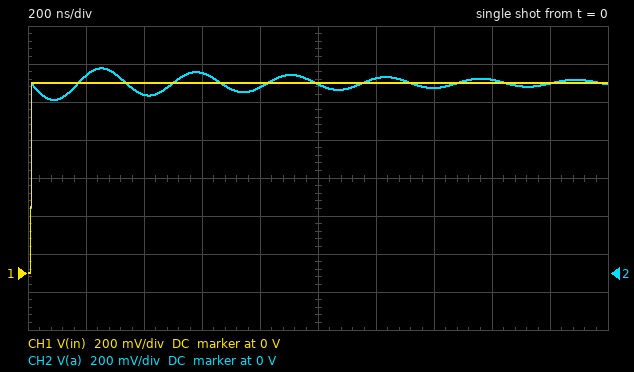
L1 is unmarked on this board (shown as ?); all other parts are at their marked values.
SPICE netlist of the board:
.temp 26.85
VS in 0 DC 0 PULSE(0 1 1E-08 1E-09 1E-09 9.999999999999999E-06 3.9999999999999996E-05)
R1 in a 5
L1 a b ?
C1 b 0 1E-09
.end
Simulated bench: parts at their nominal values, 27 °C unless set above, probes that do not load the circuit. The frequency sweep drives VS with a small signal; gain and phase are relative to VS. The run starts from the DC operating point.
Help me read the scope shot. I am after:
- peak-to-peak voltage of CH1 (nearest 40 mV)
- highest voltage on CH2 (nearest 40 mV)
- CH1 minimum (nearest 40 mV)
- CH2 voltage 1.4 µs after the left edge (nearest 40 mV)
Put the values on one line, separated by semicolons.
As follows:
1.00 V; 1.08 V; 0 V; 960 mV
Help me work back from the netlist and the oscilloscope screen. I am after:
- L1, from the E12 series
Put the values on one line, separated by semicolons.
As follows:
2.7 µH
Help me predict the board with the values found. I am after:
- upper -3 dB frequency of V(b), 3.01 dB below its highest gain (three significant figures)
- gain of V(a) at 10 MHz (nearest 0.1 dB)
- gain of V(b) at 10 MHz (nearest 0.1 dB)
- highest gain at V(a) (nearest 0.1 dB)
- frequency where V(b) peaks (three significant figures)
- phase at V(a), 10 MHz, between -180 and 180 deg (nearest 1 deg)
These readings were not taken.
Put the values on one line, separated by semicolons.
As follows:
3.20 MHz; 0 dB; -19.7 dB; 0 dB; 3.06 MHz; 2 deg
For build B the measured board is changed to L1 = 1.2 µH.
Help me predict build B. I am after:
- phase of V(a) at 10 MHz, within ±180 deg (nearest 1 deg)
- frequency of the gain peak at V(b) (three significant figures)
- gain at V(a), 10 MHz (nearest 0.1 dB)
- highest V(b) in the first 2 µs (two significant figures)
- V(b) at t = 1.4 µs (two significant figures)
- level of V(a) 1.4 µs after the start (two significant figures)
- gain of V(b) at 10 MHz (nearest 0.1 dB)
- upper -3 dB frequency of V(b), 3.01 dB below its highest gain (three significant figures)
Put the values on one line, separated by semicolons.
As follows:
5 deg; 4.57 MHz; 0 dB; 1.8 V; 1.0 V; 990 mV; -11.5 dB; 4.89 MHz
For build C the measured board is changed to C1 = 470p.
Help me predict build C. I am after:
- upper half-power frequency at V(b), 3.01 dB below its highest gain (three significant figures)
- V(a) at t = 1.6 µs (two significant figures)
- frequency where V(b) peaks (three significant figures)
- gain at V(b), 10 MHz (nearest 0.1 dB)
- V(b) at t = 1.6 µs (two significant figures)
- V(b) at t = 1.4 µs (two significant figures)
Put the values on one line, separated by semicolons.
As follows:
4.61 MHz; 990 mV; 4.46 MHz; -12.1 dB; 810 mV; 910 mV
